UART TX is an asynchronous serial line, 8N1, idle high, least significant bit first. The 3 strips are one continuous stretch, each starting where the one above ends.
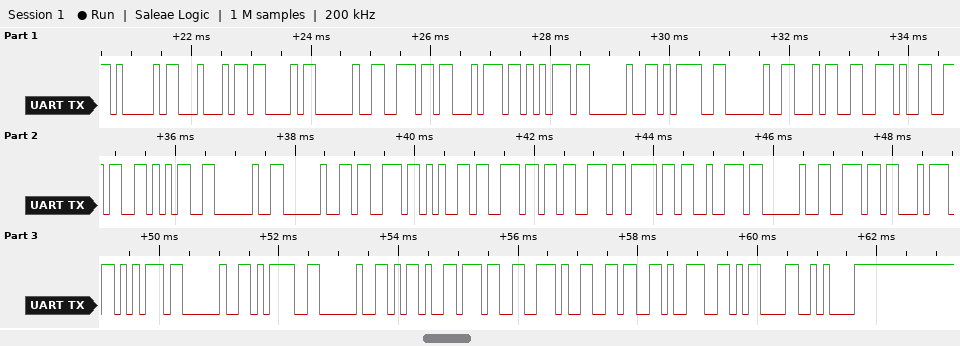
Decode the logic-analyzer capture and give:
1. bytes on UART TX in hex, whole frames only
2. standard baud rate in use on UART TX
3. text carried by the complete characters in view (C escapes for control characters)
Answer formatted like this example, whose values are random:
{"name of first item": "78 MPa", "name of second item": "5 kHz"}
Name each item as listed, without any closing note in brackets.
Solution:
{"bytes on UART TX in hex, whole frames only": "41 44 43 20 6E 74 75 20 3D 20 34 2E 36 35 20 20 73 65 6E 73 6F 72 20 6E 74 75 20 3D 20 2D 37 2E 36 39 0D 0A", "standard baud rate in use on UART TX": "9600 baud", "text carried by the complete characters in view": "\"ADC ntu = 4.65  sensor ntu = -7.69\\r\\n\""}
